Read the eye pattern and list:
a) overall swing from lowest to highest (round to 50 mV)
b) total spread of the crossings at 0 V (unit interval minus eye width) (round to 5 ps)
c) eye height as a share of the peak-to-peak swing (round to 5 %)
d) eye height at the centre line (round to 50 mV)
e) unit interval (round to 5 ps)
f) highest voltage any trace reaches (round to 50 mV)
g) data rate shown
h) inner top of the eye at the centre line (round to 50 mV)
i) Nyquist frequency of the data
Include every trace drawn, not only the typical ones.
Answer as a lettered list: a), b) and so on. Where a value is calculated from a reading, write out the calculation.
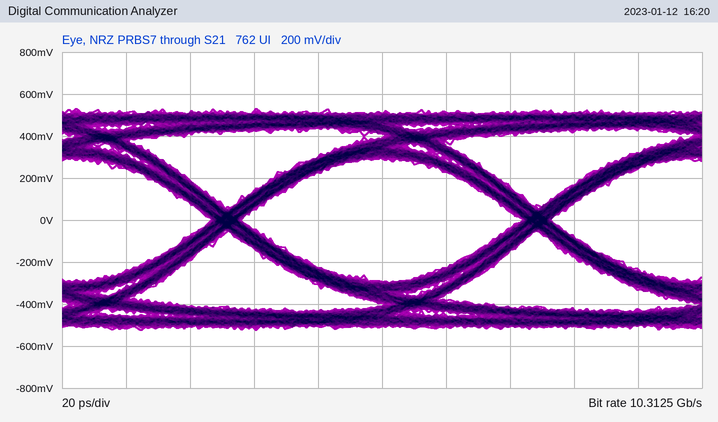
a) 1.05 V
b) 10 ps
c) 600 mV / 1.05 V ≈ 57.1 %, so 55 % to the nearest 5 %
d) 600 mV
e) 95 ps
f) 550 mV
g) 10.3125 Gb/s
h) 300 mV
i) 5.15625 GHz
